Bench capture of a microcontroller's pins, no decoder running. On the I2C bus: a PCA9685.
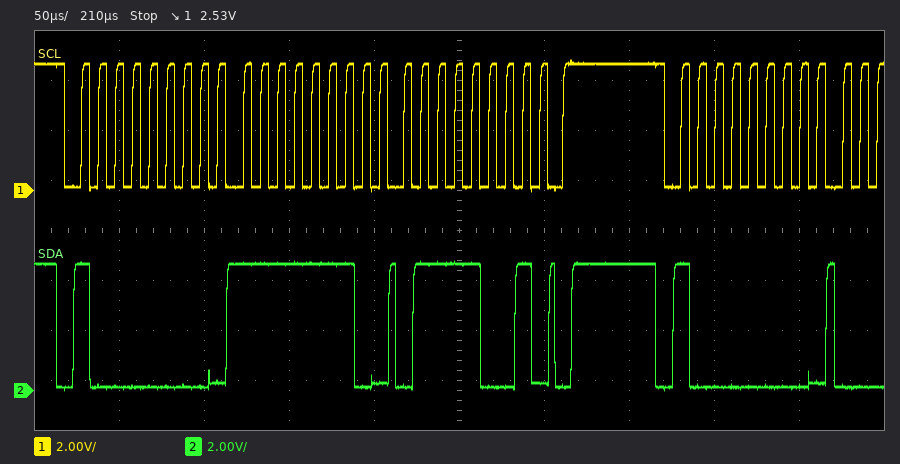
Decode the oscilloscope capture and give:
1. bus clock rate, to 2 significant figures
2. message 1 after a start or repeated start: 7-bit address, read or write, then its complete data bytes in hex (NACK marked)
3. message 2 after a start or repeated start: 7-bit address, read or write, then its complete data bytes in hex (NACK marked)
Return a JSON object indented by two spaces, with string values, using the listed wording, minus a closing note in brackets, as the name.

{
  "bus clock rate, to 2 significant figures": "100 kHz",
  "message 1 after a start or repeated start: 7-bit address, read or write, then its complete data bytes in hex": "0x40 write: FE 79",
  "message 2 after a start or repeated start: 7-bit address, read or write, then its complete data bytes in hex": "0x40 write"
}
